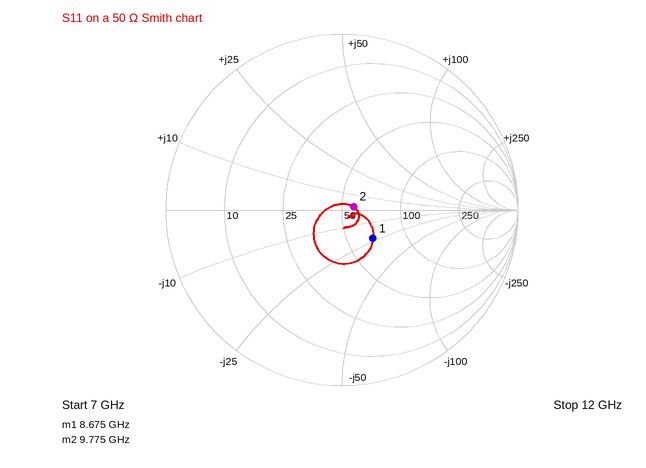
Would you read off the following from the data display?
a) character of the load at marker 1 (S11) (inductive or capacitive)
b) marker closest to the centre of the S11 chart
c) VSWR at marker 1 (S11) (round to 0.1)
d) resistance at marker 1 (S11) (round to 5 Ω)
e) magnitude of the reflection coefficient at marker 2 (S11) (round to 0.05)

capacitive
marker 2
1.6
65 Ω
0.05
